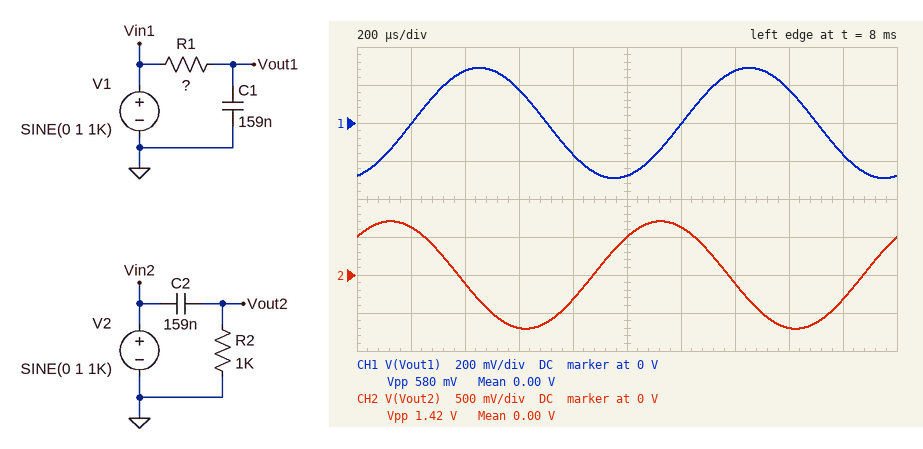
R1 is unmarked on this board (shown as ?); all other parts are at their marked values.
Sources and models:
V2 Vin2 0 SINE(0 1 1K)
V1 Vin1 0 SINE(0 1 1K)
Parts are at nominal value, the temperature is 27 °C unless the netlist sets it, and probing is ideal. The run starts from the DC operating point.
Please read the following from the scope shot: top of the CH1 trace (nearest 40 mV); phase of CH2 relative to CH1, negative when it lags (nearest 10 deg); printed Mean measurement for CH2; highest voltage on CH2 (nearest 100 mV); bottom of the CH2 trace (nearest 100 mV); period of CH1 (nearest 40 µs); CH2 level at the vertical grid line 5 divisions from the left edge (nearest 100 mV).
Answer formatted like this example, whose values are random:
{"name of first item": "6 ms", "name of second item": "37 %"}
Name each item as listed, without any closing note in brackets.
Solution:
{"top of the CH1 trace": "280 mV", "phase of CH2 relative to CH1, negative when it lags": "120 deg", "printed Mean measurement for CH2": "0.00 V", "highest voltage on CH2": "700 mV", "bottom of the CH2 trace": "-700 mV", "period of CH1": "1.00 ms", "CH2 level at the vertical grid line 5 divisions from the left edge": "500 mV"}
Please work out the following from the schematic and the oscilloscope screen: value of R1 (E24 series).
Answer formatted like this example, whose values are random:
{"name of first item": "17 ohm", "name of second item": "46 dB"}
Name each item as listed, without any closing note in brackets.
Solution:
{"value of R1": "3.3 kΩ"}
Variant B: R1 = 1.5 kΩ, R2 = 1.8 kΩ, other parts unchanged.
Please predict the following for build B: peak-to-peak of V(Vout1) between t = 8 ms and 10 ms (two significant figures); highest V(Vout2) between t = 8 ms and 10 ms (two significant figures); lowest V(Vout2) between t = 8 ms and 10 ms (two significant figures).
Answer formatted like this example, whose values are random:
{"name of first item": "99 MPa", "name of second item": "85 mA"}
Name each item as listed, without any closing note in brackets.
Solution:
{"peak-to-peak of V(Vout1) between t = 8 ms and 10 ms": "1.1 V", "highest V(Vout2) between t = 8 ms and 10 ms": "870 mV", "lowest V(Vout2) between t = 8 ms and 10 ms": "-870 mV"}
